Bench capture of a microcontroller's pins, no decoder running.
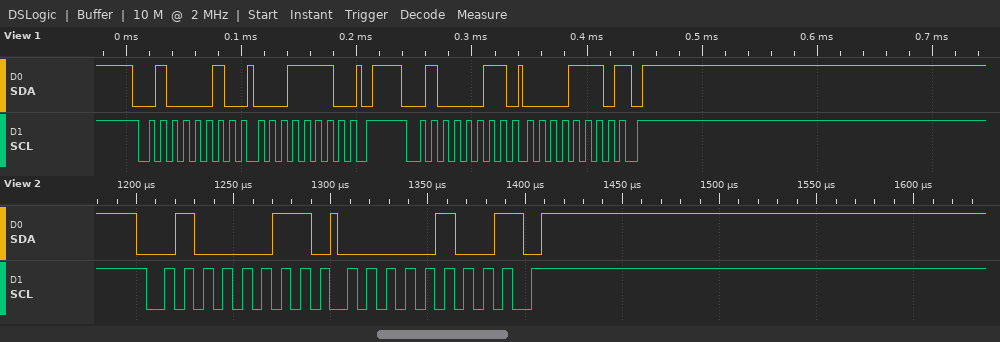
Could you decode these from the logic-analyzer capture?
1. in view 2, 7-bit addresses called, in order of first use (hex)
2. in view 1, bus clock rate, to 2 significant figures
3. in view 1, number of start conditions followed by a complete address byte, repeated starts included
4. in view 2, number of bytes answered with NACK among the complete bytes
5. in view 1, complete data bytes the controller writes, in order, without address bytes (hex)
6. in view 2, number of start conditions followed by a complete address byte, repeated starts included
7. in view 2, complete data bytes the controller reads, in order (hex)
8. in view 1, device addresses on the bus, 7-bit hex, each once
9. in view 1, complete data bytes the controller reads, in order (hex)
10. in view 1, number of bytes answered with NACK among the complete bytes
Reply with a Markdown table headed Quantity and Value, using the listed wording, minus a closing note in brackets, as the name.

| Quantity | Value |
|---|---|
| in view 2, 7-bit addresses called, in order of first use | 0x21 |
| in view 1, bus clock rate, to 2 significant figures | 100 kHz |
| in view 1, number of start conditions followed by a complete address byte, repeated starts included | 2 |
| in view 2, number of bytes answered with NACK among the complete bytes | 1 |
| in view 1, complete data bytes the controller writes, in order, without address bytes | 1E |
| in view 2, number of start conditions followed by a complete address byte, repeated starts included | 1 |
| in view 2, complete data bytes the controller reads, in order | 04 |
| in view 1, device addresses on the bus, 7-bit hex, each once | 0x21 |
| in view 1, complete data bytes the controller reads, in order | 0E |
| in view 1, number of bytes answered with NACK among the complete bytes | 1 |
